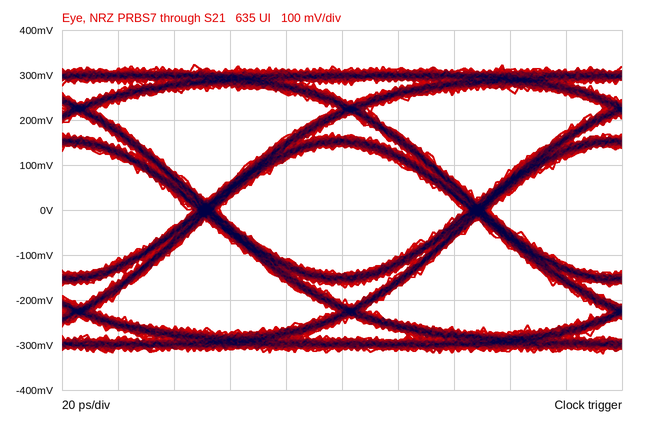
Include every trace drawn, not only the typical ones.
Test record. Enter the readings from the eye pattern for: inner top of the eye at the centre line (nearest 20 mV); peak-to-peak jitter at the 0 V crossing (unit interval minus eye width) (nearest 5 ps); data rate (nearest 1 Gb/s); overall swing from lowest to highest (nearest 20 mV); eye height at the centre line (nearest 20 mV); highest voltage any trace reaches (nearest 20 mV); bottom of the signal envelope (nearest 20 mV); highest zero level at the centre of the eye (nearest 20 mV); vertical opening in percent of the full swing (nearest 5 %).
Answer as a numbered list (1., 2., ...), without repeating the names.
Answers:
1. 140 mV
2. 10 ps
3. 10 Gb/s
4. 640 mV
5. 280 mV
6. 320 mV
7. -320 mV
8. -140 mV
9. 45 %
